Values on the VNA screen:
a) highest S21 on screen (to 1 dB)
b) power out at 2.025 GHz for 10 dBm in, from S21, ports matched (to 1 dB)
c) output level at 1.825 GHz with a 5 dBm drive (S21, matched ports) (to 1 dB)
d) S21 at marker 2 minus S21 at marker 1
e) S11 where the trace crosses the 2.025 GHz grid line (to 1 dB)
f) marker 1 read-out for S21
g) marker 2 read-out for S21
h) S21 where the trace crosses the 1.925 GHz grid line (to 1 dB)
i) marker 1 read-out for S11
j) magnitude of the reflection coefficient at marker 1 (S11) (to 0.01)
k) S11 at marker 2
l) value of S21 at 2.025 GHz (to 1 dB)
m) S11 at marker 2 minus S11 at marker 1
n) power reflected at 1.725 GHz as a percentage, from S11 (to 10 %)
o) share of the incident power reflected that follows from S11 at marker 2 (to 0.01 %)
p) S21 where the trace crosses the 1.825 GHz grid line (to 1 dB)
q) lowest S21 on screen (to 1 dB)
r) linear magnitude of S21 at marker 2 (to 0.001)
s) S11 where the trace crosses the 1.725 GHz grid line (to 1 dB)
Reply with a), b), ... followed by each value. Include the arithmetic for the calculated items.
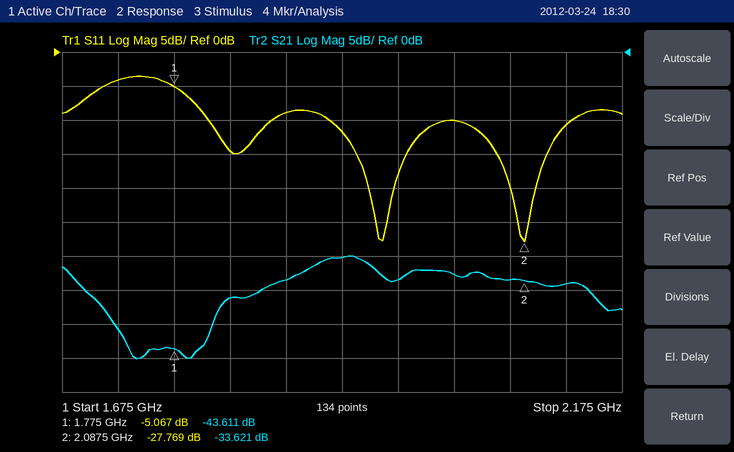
a) -30 dB
b) 10 dBm + (-33 dB) = -23 dBm
c) 5 dBm + (-36 dB) = -31 dBm
d) -33.621 − (-43.611) = 9.990 dB
e) -10 dB
f) -43.611 dB
g) -33.621 dB
h) -30 dB
i) -5.067 dB
j) 10^(-5.067/20) ≈ 0.56
k) -27.769 dB
l) -33 dB
m) -27.769 − (-5.067) = -22.702 dB
n) 10^(-4/10) ≈ 40 %
o) 10^(-27.769/10) ≈ 0.17 %
p) -36 dB
q) -45 dB
r) 10^(-33.621/20) ≈ 0.021
s) -4 dB
